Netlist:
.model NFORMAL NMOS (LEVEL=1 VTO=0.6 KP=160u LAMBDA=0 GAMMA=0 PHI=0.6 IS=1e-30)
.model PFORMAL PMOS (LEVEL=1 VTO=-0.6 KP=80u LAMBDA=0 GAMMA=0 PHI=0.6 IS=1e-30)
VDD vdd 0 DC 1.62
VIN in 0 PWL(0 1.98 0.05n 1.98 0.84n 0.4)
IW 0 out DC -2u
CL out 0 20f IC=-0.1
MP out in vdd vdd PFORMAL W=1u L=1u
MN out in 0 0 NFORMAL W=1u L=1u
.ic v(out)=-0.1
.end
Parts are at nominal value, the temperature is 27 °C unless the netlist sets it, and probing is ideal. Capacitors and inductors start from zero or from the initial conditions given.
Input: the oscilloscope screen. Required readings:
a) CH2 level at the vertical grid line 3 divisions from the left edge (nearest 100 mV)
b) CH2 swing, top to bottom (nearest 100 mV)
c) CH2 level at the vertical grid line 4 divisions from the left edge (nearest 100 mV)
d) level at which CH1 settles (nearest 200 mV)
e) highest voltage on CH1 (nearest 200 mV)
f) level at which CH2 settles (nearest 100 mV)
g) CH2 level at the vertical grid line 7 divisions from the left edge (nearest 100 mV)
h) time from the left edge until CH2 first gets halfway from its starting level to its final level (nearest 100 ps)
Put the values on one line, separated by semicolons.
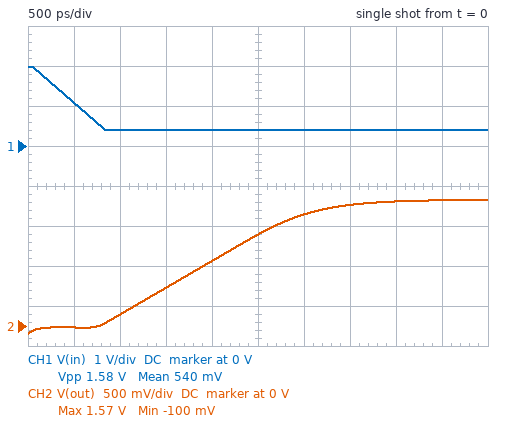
500 mV; 1.7 V; 800 mV; 400 mV; 2.0 V; 1.6 V; 1.5 V; 1.9 ns
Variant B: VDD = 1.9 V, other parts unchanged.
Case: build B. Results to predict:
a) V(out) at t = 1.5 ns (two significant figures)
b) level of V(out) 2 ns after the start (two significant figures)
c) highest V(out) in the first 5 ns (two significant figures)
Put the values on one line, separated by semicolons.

1.2 V; 1.7 V; 1.9 V
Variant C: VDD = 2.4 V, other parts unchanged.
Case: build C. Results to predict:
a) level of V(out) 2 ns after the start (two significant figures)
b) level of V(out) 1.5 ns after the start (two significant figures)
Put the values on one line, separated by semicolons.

2.4 V; 2.3 V
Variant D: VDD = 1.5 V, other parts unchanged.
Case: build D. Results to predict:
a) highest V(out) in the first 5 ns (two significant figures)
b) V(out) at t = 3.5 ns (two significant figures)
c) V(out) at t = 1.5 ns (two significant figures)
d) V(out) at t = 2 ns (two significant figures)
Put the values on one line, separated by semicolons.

1.4 V; 1.1 V; 260 mV; 460 mV
